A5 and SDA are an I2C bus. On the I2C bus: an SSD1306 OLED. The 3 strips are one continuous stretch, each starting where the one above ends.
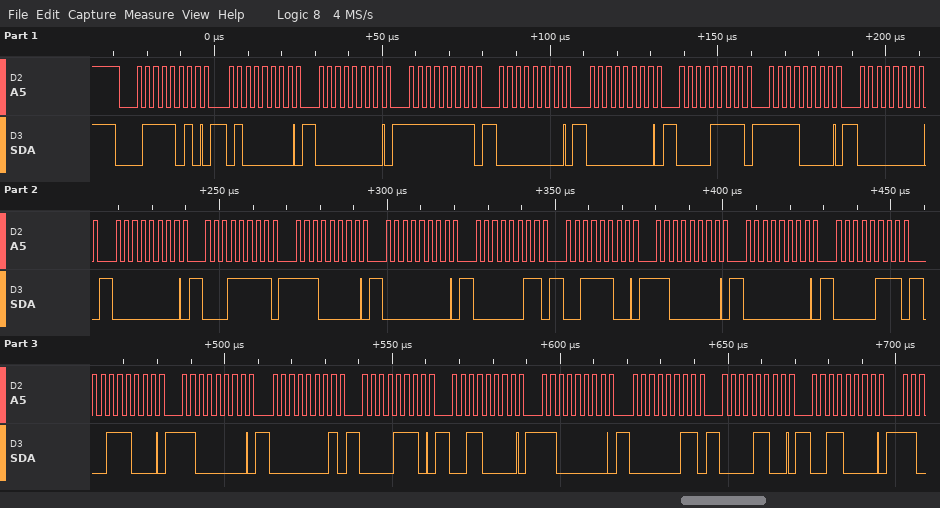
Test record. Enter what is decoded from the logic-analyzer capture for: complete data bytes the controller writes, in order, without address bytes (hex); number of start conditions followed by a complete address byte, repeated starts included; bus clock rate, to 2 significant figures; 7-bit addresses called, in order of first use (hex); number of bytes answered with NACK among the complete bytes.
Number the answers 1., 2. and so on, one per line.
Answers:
1. 40 00 FF 00 00 0F F0 00 00 1F E0 00 03 3C C0 00 07 38 C0 01 0E 30 C0 03 0C 30
2. 1
3. 400 kHz
4. 0x3D
5. 0
